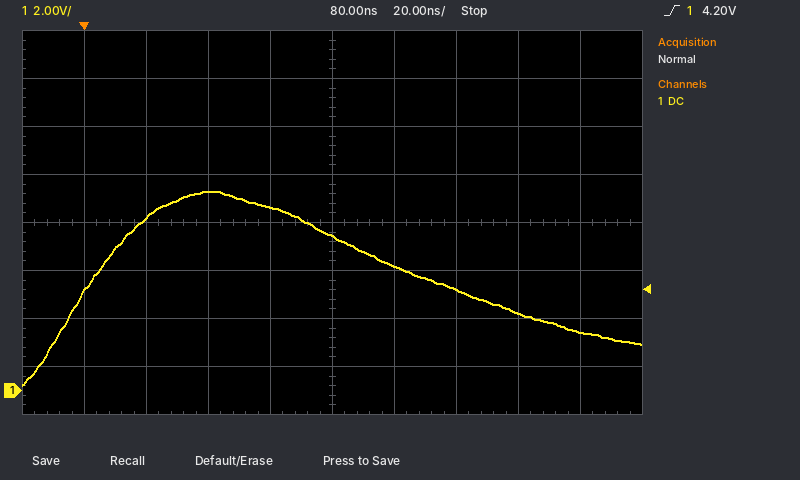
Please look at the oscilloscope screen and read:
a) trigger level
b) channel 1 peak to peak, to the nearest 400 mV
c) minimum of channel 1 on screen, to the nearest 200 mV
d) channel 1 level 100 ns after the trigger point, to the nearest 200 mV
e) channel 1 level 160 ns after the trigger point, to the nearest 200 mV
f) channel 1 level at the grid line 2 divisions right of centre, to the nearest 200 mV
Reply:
4.20 V
8.0 V
200 mV
5.2 V
2.4 V
4.2 V
